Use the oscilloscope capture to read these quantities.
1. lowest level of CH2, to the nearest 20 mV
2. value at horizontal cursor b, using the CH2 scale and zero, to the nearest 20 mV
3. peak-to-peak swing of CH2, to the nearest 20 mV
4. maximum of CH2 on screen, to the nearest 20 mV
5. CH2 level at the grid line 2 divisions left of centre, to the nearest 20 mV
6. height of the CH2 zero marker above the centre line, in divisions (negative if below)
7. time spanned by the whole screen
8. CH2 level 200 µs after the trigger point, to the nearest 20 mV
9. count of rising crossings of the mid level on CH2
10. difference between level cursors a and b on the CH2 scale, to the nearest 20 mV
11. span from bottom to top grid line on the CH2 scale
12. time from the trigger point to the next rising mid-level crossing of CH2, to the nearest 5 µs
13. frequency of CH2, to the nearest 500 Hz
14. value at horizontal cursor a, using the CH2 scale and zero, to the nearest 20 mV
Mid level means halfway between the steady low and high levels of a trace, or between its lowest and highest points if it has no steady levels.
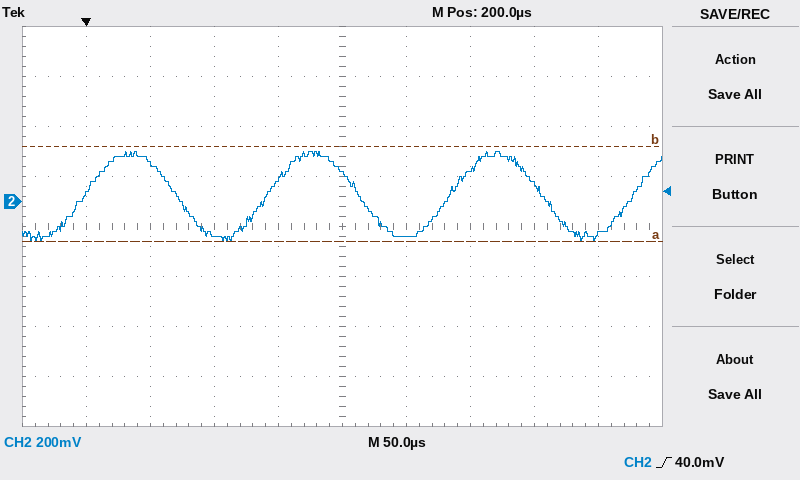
-160 mV
220 mV
360 mV
200 mV
-140 mV
+0.5 div
500 µs
120 mV
4
380 mV
1.6 V
140 µs
7.0 kHz
-160 mV
